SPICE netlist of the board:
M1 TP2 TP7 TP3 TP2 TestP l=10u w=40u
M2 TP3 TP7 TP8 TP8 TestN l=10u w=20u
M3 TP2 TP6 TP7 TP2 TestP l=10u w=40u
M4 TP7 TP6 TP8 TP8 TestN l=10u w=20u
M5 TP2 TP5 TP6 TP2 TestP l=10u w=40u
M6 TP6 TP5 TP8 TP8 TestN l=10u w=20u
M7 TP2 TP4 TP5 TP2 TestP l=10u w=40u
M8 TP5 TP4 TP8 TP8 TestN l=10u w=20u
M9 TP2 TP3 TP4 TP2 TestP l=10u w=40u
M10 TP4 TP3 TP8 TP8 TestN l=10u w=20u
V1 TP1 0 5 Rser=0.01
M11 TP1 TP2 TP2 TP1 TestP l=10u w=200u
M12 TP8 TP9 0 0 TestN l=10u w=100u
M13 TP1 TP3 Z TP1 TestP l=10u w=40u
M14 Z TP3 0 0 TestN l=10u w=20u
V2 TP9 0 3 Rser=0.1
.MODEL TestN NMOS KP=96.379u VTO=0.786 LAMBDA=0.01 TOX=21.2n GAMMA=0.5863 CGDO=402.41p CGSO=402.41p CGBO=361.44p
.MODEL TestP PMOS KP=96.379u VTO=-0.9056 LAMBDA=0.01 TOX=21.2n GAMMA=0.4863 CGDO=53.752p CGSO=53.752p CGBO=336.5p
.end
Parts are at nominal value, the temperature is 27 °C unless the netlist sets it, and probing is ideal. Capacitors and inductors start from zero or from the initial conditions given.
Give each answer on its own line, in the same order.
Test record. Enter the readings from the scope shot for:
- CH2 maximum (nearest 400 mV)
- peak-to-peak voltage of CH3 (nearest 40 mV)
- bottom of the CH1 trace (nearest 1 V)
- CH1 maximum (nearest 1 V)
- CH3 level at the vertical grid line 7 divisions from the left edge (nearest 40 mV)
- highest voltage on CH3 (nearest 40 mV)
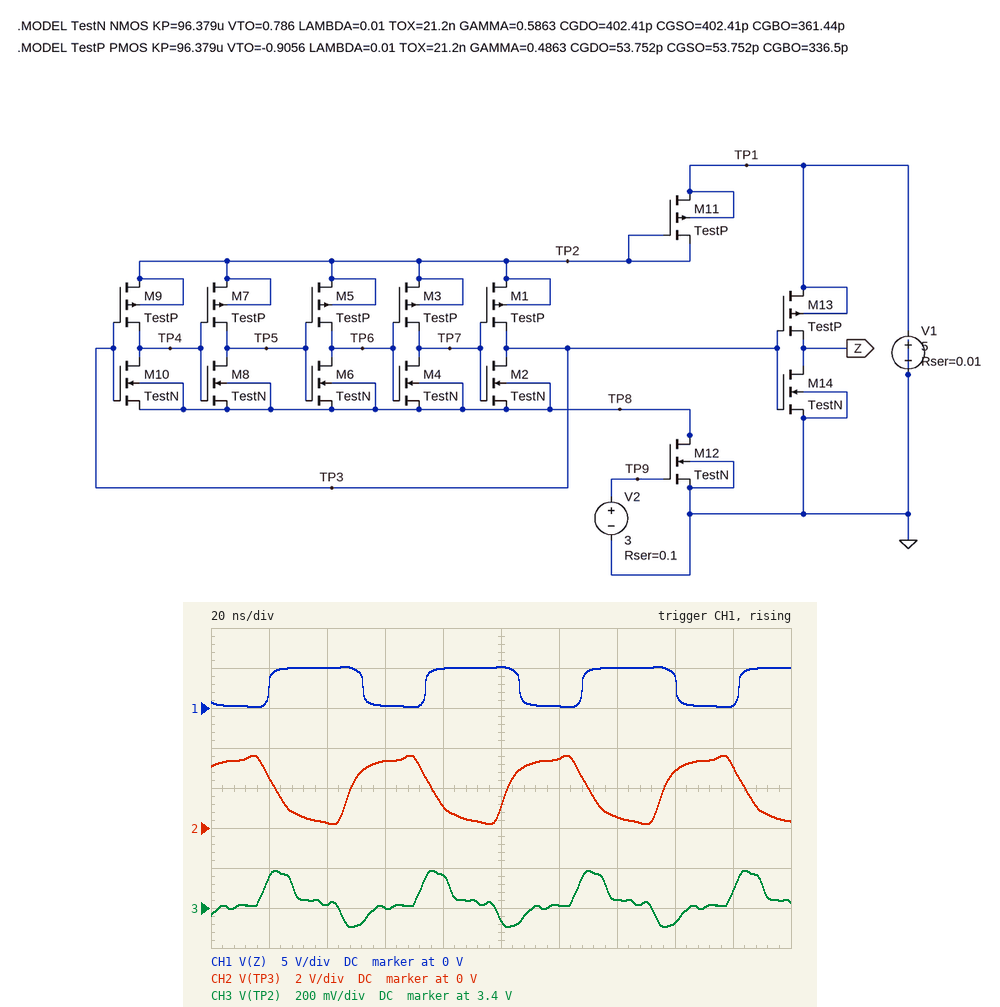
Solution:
3.6 V
280 mV
0 V
5 V
3.44 V
3.60 V
